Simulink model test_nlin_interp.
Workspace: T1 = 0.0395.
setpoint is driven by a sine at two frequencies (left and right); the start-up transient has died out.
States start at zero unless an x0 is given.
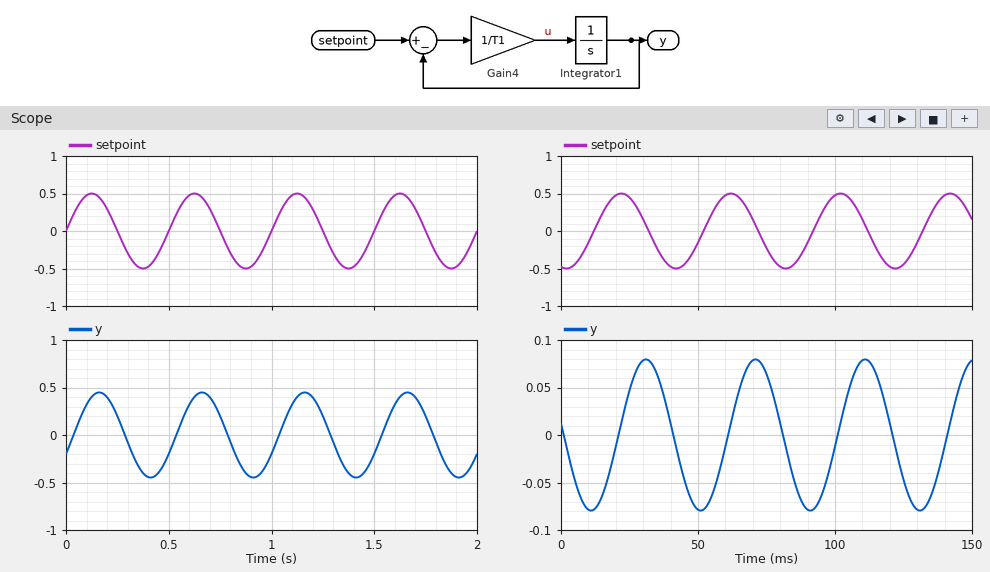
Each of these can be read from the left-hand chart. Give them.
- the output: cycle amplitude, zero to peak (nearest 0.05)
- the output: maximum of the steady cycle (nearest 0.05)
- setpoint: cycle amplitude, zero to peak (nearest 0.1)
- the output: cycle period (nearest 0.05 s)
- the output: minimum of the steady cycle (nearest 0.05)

0.45
0.45
0.5
0.50 s
-0.45
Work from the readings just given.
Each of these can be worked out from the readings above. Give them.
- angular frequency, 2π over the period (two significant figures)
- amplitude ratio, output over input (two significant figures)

13 rad/s
0.90
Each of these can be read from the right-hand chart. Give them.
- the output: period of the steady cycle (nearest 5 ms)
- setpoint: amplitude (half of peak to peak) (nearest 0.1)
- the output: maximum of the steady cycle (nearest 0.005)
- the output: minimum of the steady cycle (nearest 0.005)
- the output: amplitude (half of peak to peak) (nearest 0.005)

40 ms
0.5
0.080
-0.080
0.080
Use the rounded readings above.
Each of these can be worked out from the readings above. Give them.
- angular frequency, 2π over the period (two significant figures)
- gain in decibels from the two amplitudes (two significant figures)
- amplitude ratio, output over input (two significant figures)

0.16 rad/ms
-16 dB
0.16
